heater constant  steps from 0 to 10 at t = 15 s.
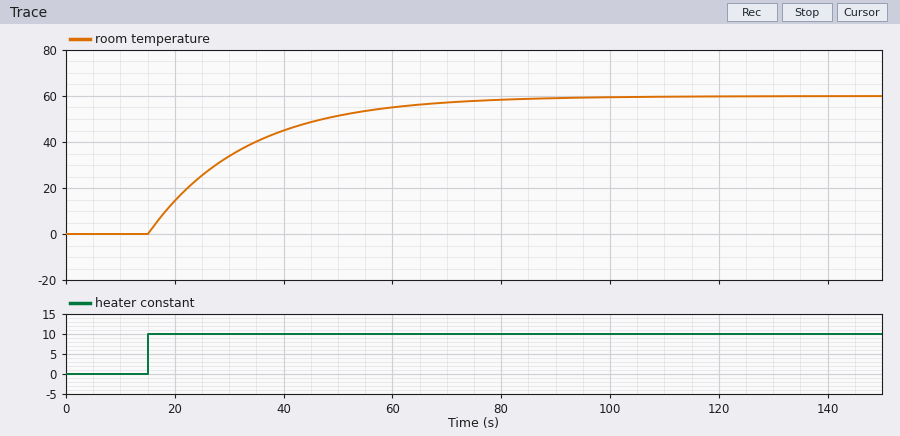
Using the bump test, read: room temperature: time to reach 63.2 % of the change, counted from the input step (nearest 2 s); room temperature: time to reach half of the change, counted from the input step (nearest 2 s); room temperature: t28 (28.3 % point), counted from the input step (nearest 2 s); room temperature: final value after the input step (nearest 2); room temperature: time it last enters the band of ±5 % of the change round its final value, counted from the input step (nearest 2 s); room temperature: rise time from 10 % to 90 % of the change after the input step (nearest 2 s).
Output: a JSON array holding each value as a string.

["18 s", "12 s", "6 s", "60", "54 s", "40 s"]
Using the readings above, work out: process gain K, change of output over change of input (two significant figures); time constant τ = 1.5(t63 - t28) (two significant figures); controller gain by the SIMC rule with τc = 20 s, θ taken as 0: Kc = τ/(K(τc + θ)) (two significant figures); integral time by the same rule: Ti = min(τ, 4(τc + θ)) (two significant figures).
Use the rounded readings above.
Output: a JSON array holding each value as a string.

["6.0", "18 s", "0.15", "18 s"]
